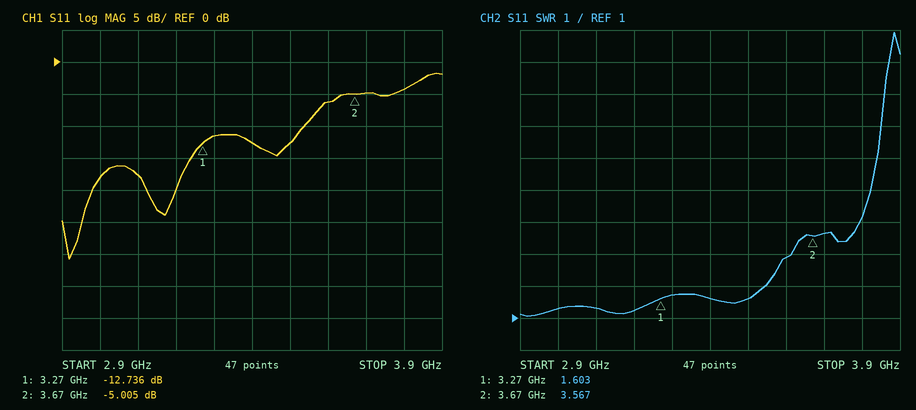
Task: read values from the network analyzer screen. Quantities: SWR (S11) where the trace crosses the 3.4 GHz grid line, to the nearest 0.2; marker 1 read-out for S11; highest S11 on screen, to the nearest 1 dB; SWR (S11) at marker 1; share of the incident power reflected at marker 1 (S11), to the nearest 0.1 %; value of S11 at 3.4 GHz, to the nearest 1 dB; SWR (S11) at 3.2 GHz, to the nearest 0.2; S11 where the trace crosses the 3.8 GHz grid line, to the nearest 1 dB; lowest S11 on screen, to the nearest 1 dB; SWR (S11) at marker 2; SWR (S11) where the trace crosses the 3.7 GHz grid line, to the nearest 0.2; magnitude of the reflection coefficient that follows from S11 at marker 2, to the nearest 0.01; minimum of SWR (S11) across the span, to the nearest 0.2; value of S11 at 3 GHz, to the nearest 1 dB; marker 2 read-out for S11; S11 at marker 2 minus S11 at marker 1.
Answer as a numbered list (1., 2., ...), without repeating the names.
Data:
1. 1.6
2. -12.736 dB
3. -2 dB
4. 1.603
5. 5.3 %
6. -13 dB
7. 1.2
8. -4 dB
9. -31 dB
10. 3.567
11. 3.6
12. 0.56
13. 1.0
14. -18 dB
15. -5.005 dB
16. 7.731 dB
